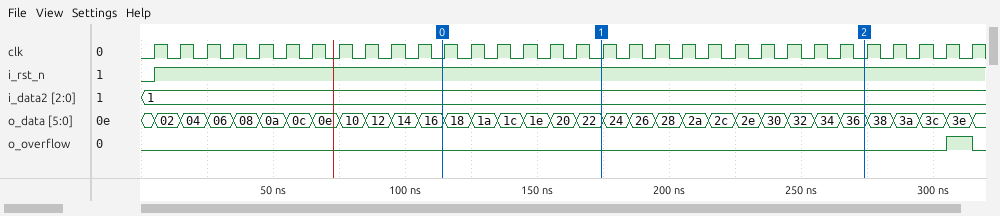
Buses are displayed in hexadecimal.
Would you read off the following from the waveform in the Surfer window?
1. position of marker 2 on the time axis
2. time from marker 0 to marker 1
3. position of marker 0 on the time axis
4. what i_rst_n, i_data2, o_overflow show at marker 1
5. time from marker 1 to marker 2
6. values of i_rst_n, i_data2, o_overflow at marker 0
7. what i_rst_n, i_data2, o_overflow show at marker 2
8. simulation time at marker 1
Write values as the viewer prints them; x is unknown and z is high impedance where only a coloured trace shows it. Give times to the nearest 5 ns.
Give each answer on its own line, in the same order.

275 ns
60 ns
115 ns
i_rst_n=1, i_data2=1, o_overflow=0
100 ns
i_rst_n=1, i_data2=1, o_overflow=0
i_rst_n=1, i_data2=1, o_overflow=0
175 ns
